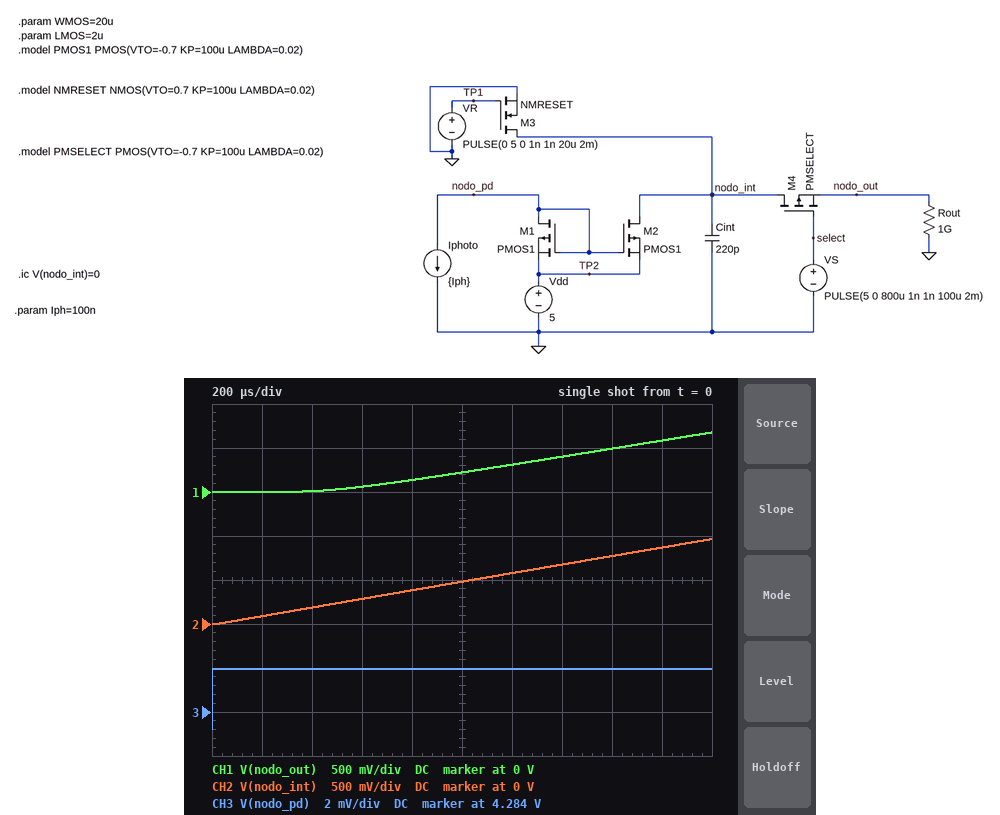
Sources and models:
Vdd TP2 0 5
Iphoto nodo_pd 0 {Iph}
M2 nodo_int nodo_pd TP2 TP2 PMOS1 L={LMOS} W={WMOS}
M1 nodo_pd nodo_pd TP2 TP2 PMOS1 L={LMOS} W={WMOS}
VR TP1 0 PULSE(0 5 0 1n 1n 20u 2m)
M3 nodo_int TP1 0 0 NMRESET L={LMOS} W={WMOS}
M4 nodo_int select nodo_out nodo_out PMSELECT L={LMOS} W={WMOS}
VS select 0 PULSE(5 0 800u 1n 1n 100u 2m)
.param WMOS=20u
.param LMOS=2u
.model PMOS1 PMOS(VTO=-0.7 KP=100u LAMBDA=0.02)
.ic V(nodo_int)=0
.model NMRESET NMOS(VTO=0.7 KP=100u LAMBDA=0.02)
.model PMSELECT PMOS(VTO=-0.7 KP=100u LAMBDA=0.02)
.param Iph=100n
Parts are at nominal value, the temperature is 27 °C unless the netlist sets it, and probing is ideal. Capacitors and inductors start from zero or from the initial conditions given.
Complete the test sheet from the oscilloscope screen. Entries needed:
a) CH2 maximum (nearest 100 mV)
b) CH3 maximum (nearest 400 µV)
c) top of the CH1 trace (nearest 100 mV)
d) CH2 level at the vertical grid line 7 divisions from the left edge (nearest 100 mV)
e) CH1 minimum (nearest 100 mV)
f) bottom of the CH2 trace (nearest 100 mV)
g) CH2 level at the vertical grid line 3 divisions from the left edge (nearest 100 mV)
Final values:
1.0 V
4.2860 V
700 mV
700 mV
0 V
0 V
300 mV
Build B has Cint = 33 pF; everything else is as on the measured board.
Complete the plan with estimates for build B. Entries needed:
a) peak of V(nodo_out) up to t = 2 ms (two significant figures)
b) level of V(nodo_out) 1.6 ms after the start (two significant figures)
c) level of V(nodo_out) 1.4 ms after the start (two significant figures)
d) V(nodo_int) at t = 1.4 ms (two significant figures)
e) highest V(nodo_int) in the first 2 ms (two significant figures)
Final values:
4.7 V
4.5 V
3.9 V
4.3 V
5.0 V
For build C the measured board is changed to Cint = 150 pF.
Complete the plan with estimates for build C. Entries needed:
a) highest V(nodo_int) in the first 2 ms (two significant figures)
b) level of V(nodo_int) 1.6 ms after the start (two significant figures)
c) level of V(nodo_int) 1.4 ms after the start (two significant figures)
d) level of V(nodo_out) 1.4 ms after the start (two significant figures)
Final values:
1.4 V
1.1 V
990 mV
700 mV
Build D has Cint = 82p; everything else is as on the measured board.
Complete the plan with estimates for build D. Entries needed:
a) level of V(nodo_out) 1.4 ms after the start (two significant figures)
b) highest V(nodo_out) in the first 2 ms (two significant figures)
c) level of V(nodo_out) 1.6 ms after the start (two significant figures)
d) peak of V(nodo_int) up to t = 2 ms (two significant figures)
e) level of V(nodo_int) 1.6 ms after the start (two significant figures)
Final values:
1.5 V
2.2 V
1.7 V
2.5 V
2.0 V
